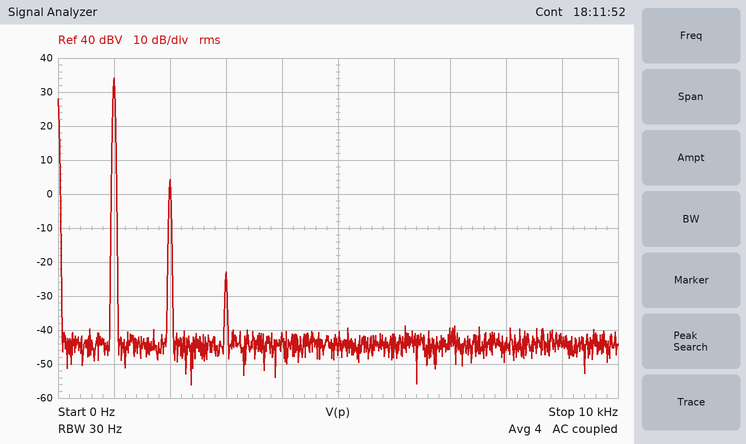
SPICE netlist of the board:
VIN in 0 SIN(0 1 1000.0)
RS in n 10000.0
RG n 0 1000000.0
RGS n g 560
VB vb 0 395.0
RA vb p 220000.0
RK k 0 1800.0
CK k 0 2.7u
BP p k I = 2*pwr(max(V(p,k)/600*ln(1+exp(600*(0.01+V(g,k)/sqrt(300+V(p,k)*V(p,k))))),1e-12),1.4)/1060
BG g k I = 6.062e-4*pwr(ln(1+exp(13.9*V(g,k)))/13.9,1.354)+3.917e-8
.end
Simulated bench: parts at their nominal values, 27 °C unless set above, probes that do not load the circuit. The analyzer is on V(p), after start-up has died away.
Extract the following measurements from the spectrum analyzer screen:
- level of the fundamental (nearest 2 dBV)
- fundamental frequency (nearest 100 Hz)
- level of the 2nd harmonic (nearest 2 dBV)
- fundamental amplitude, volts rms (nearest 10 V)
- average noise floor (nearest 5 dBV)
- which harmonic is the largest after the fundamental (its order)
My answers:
34 dBV
1.0 kHz
4 dBV
50 V
-45 dBV
2
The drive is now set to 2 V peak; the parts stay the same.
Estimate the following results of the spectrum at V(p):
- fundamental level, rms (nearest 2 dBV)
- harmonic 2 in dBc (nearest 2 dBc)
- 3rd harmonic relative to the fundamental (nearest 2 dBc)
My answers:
40 dBV
-34 dBc
-28 dBc
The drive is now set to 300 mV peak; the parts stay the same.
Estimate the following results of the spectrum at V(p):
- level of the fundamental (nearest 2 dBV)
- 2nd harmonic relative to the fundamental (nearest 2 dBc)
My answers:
24 dBV
-40 dBc
